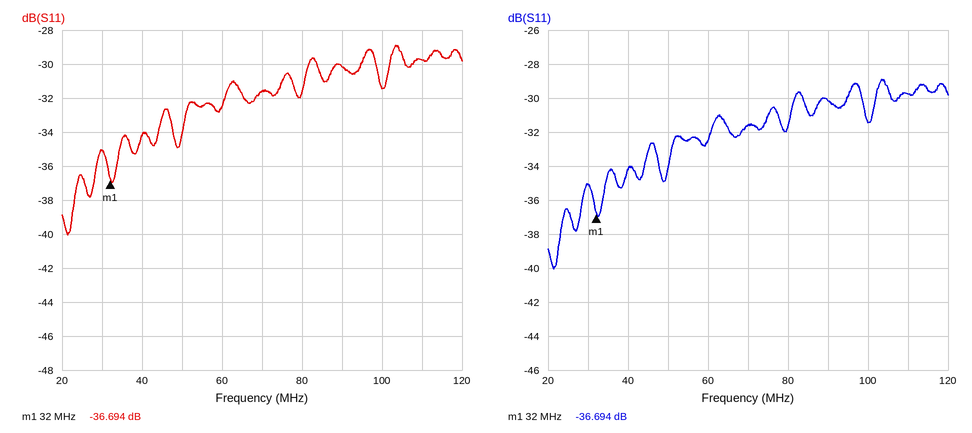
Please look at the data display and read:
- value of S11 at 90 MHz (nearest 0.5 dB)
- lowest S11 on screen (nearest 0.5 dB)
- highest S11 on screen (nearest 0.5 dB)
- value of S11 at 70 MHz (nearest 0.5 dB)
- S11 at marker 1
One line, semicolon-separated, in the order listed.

-30.0 dB; -40.0 dB; -29.0 dB; -31.5 dB; -36.694 dB
